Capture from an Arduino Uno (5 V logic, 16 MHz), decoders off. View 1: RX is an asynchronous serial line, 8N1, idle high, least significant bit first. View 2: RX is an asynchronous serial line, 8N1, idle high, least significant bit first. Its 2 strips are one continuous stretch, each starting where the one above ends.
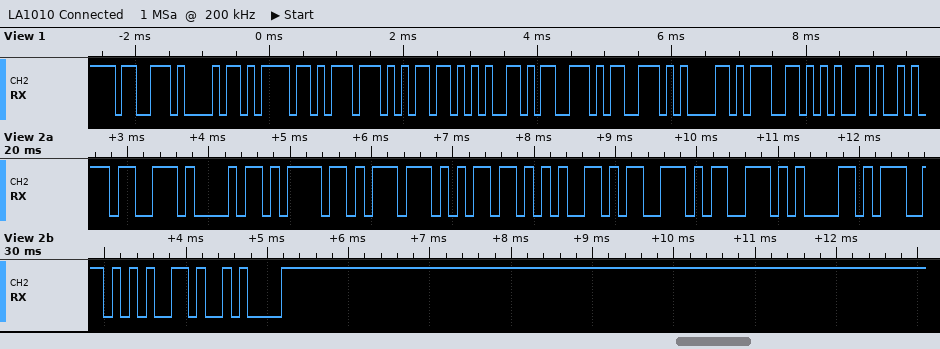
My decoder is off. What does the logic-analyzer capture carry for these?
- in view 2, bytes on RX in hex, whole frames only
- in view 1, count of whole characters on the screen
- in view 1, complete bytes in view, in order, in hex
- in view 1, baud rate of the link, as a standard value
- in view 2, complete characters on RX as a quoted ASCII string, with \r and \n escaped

73 68 6F 77 6D 65 73 73 61 67 65 0A
11
0x73 0x68 0x6F 0x77 0x6D 0x65 0x73 0x73 0x61 0x67 0x65
9600 baud
"showmessage\n"
